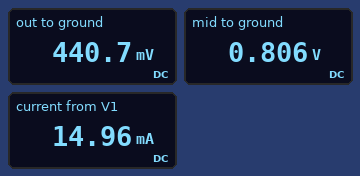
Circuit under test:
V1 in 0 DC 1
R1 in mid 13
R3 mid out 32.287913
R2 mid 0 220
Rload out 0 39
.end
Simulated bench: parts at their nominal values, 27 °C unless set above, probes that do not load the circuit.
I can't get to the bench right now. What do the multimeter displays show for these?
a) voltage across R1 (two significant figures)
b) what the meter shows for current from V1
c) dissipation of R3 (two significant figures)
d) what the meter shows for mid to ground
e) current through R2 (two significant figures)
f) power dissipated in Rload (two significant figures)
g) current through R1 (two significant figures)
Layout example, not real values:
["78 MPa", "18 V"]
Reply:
["190 mV", "14.96 mA", "4.1 mW", "0.806 V", "3.7 mA", "5.0 mW", "15 mA"]
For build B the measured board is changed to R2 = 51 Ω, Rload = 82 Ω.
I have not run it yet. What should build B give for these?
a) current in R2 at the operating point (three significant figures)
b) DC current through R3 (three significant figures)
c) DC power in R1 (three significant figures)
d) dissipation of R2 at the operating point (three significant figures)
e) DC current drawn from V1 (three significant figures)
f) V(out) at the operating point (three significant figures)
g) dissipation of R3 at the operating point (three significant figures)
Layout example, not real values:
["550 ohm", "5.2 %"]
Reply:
["14.3 mA", "6.39 mA", "5.58 mW", "10.5 mW", "20.7 mA", "524 mV", "1.32 mW"]
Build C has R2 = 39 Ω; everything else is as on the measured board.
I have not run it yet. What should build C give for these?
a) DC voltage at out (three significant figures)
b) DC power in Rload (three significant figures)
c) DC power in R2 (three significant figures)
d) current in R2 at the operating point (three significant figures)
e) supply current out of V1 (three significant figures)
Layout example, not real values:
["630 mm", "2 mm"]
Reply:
["361 mV", "3.34 mW", "11.2 mW", "16.9 mA", "26.2 mA"]
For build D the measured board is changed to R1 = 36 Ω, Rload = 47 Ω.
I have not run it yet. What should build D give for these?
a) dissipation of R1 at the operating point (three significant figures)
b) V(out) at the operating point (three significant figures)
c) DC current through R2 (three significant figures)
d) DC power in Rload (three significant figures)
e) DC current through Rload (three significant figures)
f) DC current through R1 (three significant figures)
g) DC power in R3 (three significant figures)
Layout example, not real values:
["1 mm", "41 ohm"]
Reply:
["4.05 mW", "366 mV", "2.81 mA", "2.86 mW", "7.80 mA", "10.6 mA", "1.96 mW"]
